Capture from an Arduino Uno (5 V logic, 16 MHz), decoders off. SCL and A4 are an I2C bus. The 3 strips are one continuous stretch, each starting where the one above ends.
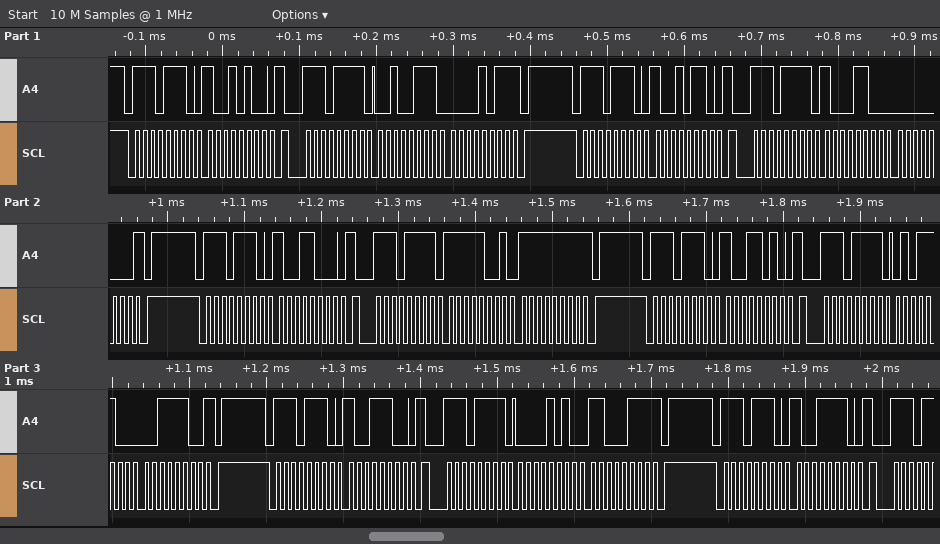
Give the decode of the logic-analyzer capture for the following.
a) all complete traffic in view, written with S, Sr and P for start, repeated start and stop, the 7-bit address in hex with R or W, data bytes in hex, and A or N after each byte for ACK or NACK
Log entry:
S 77W A 94 A Sr 77R A 27 A 0B N P S 77W A 96 A Sr 77R A 8C A 00 N P S 77W A 98 A Sr 77R A F9 A FF N P S 77W A 9A A Sr 77R A 5C A 3C N P S 77W A 9C A Sr 77R A 0A A C7 N P S 77W A 9E A
